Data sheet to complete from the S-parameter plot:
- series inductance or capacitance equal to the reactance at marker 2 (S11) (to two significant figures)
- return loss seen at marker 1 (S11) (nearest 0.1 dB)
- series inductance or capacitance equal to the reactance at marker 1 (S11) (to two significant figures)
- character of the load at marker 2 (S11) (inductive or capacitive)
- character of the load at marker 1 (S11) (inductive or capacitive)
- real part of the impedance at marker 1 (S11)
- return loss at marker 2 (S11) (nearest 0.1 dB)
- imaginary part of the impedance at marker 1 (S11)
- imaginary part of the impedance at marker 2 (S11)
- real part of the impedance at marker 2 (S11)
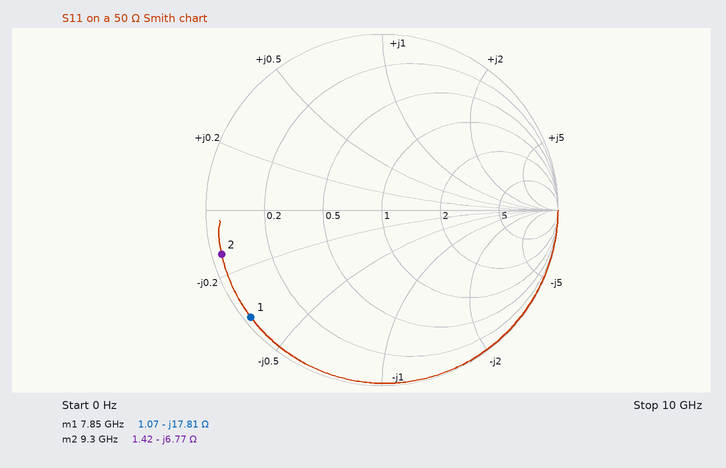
2.5 pF
0.3 dB
1.1 pF
capacitive
capacitive
1.07 Ω
0.5 dB
-17.81 Ω
-6.77 Ω
1.42 Ω
